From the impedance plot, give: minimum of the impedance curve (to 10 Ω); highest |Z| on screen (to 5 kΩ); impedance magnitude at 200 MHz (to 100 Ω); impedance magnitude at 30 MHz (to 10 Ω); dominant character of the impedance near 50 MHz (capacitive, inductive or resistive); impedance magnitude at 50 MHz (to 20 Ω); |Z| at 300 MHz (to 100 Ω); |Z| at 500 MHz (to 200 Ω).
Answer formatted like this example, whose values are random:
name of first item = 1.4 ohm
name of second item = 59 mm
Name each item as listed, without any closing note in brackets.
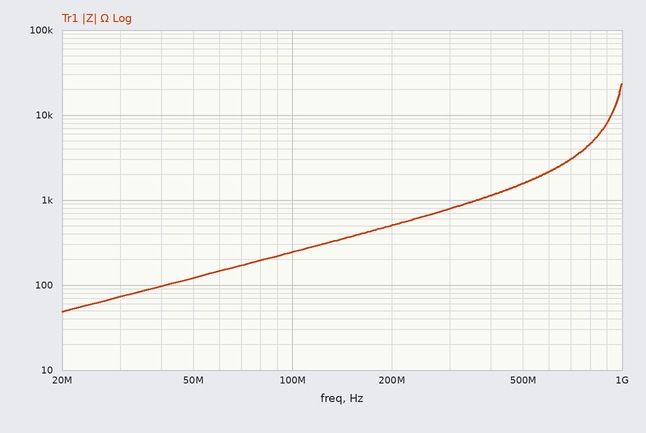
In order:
minimum of the impedance curve = 50 Ω
highest |Z| on screen = 25 kΩ
impedance magnitude at 200 MHz = 500 Ω
impedance magnitude at 30 MHz = 70 Ω
dominant character of the impedance near 50 MHz = inductive
impedance magnitude at 50 MHz = 120 Ω
|Z| at 300 MHz = 800 Ω
|Z| at 500 MHz = 1.6 kΩ
